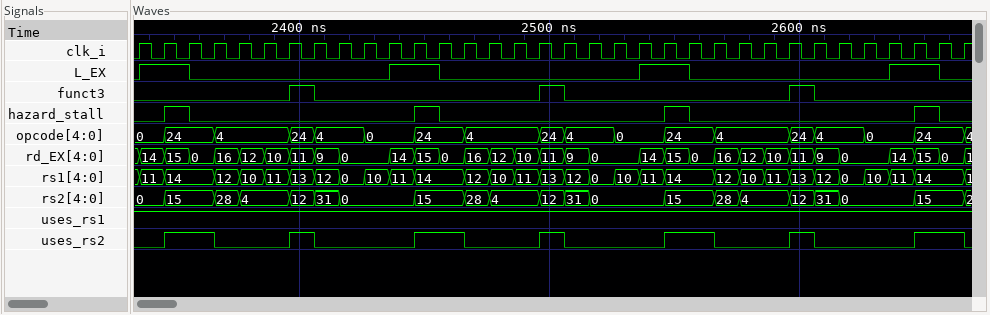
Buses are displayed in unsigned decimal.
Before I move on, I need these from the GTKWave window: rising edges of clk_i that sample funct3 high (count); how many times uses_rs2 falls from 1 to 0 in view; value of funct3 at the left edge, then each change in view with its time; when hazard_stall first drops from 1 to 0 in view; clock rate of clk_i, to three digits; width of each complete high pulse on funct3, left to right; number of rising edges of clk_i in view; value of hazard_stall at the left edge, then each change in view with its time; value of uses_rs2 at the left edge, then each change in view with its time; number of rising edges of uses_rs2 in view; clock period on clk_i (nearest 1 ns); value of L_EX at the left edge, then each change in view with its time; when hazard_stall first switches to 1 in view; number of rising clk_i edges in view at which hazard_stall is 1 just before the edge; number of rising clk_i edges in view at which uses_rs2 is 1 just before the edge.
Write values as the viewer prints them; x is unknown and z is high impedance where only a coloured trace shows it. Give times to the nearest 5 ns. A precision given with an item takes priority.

3
7
0, 1 at 2395 ns, 0 at 2405 ns, 1 at 2495 ns, 0 at 2505 ns, 1 at 2595 ns, 0 at 2605 ns
2355 ns
100 MHz
10 ns, 10 ns, 10 ns
34
0, 1 at 2345 ns, 0 at 2355 ns, 1 at 2445 ns, 0 at 2455 ns, 1 at 2545 ns, 0 at 2555 ns, 1 at 2645 ns, 0 at 2655 ns
0, 1 at 2345 ns, 0 at 2365 ns, 1 at 2395 ns, 0 at 2405 ns, 1 at 2445 ns, 0 at 2465 ns, 1 at 2495 ns, 0 at 2505 ns, 1 at 2545 ns, 0 at 2565 ns, 1 at 2595 ns, 0 at 2605 ns, 1 at 2645 ns, 0 at 2665 ns
7
10 ns
0, 1 at 2335 ns, 0 at 2355 ns, 1 at 2435 ns, 0 at 2455 ns, 1 at 2535 ns, 0 at 2555 ns, 1 at 2635 ns, 0 at 2655 ns
2345 ns
4
11
